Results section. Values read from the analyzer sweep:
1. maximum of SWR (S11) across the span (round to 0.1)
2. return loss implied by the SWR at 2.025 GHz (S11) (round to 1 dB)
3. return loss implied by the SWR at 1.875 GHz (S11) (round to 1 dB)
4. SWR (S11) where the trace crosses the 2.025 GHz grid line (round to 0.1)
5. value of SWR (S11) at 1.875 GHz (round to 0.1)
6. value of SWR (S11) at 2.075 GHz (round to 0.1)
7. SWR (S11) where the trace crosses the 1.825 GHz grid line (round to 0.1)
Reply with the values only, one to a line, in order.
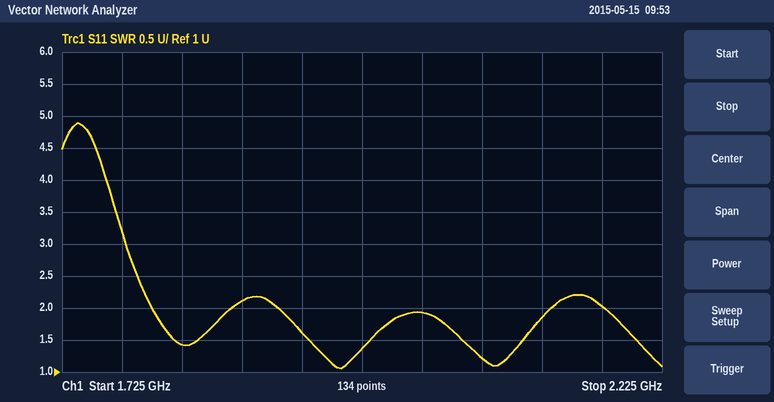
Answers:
4.9
10 dB
9 dB
1.9
2.1
1.2
1.4
